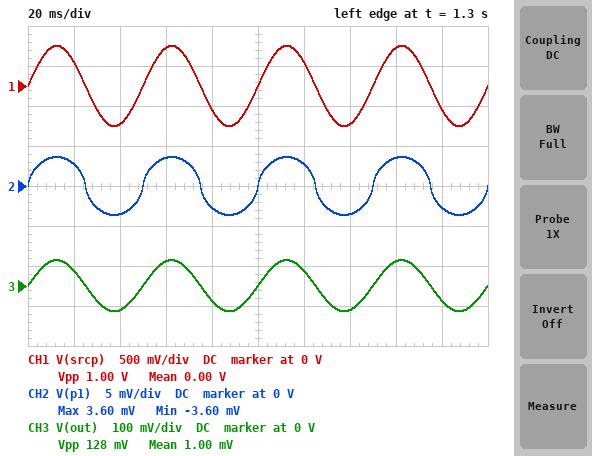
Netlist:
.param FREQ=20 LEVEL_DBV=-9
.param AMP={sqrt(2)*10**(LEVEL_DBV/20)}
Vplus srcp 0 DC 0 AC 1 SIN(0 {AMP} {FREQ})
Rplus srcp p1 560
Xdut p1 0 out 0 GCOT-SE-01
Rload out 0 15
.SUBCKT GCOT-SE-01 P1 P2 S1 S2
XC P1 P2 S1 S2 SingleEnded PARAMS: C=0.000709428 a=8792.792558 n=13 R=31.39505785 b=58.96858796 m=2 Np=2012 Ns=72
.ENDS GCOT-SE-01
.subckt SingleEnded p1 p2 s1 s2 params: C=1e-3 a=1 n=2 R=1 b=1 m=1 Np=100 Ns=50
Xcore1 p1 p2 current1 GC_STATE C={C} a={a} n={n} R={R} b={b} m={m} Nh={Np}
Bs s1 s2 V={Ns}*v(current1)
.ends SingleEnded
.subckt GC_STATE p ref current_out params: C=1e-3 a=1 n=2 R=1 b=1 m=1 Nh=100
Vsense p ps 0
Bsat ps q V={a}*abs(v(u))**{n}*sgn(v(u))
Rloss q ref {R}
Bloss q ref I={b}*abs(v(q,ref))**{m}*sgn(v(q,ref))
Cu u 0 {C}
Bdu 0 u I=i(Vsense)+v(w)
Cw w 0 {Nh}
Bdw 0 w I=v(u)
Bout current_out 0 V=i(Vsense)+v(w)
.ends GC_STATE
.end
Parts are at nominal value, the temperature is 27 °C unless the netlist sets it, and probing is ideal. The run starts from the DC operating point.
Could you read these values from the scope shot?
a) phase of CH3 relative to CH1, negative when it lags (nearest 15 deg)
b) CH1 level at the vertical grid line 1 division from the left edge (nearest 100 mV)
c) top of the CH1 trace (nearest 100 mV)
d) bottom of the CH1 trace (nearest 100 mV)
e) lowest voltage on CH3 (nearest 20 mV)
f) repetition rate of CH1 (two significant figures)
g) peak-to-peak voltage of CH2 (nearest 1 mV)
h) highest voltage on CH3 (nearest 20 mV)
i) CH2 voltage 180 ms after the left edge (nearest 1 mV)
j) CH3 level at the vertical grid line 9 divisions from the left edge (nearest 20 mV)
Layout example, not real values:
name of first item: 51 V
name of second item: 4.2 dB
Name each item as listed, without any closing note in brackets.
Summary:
phase of CH3 relative to CH1, negative when it lags: 0 deg
CH1 level at the vertical grid line 1 division from the left edge: 300 mV
top of the CH1 trace: 500 mV
bottom of the CH1 trace: -500 mV
lowest voltage on CH3: -60 mV
repetition rate of CH1: 20 Hz
peak-to-peak voltage of CH2: 7 mV
highest voltage on CH3: 60 mV
CH2 voltage 180 ms after the left edge: -3 mV
CH3 level at the vertical grid line 9 divisions from the left edge: -40 mV
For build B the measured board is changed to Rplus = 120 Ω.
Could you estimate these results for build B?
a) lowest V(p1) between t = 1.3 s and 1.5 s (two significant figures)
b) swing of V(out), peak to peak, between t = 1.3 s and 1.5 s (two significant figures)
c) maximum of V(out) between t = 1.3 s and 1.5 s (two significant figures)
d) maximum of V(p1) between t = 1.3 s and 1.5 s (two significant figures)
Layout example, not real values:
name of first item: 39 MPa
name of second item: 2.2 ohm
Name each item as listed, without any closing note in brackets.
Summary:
lowest V(p1) between t = 1.3 s and 1.5 s: -8.1 mV
swing of V(out), peak to peak, between t = 1.3 s and 1.5 s: 590 mV
maximum of V(out) between t = 1.3 s and 1.5 s: 300 mV
maximum of V(p1) between t = 1.3 s and 1.5 s: 8.1 mV
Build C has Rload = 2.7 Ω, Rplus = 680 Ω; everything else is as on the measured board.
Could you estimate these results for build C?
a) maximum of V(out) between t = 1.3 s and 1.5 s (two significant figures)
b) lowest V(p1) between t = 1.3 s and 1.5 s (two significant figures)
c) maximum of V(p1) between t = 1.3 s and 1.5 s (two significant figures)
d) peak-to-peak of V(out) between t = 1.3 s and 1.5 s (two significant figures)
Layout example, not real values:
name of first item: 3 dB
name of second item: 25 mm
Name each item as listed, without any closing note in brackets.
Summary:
maximum of V(out) between t = 1.3 s and 1.5 s: 53 mV
lowest V(p1) between t = 1.3 s and 1.5 s: -3.3 mV
maximum of V(p1) between t = 1.3 s and 1.5 s: 3.3 mV
peak-to-peak of V(out) between t = 1.3 s and 1.5 s: 110 mV
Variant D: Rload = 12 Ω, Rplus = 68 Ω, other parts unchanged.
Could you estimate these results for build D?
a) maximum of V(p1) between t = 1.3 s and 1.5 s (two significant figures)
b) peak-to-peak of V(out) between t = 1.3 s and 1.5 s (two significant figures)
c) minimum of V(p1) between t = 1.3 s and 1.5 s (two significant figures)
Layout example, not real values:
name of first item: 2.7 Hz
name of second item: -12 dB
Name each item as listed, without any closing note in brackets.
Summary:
maximum of V(p1) between t = 1.3 s and 1.5 s: 11 mV
peak-to-peak of V(out) between t = 1.3 s and 1.5 s: 1.0 V
minimum of V(p1) between t = 1.3 s and 1.5 s: -11 mV
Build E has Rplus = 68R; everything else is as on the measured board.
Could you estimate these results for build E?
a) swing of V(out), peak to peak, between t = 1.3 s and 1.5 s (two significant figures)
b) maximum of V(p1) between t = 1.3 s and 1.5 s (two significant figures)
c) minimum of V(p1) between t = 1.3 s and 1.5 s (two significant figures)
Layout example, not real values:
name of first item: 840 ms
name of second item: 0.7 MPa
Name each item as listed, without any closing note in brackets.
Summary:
swing of V(out), peak to peak, between t = 1.3 s and 1.5 s: 1.0 V
maximum of V(p1) between t = 1.3 s and 1.5 s: 11 mV
minimum of V(p1) between t = 1.3 s and 1.5 s: -11 mV
